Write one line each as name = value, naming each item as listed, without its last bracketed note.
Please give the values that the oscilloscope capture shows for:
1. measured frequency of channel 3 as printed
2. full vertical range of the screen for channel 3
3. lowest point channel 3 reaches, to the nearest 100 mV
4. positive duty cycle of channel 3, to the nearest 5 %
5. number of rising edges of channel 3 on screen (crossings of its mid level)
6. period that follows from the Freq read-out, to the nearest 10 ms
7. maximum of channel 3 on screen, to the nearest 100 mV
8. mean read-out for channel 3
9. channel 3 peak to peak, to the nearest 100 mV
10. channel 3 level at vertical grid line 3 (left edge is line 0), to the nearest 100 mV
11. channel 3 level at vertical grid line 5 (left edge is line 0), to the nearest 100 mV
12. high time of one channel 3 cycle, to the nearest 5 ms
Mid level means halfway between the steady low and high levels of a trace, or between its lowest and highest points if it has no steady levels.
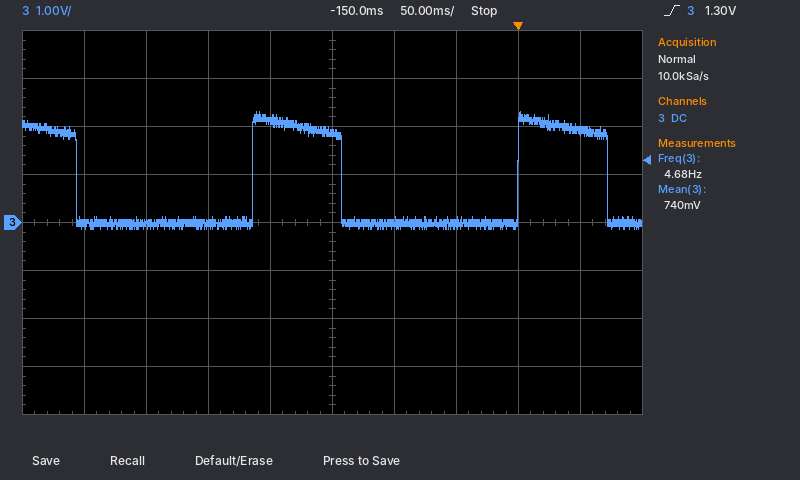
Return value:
measured frequency of channel 3 as printed = 4.68 Hz
full vertical range of the screen for channel 3 = 8 V
lowest point channel 3 reaches, to the nearest 100 mV = -100 mV
positive duty cycle of channel 3, to the nearest 5 % = 35 %
number of rising edges of channel 3 on screen = 2
period that follows from the Freq read-out, to the nearest 10 ms = 210 ms
maximum of channel 3 on screen, to the nearest 100 mV = 2.3 V
mean read-out for channel 3 = 740 mV
channel 3 peak to peak, to the nearest 100 mV = 2.4 V
channel 3 level at vertical grid line 3 (left edge is line 0), to the nearest 100 mV = 0.0 V
channel 3 level at vertical grid line 5 (left edge is line 0), to the nearest 100 mV = 1.9 V
high time of one channel 3 cycle, to the nearest 5 ms = 70 ms
